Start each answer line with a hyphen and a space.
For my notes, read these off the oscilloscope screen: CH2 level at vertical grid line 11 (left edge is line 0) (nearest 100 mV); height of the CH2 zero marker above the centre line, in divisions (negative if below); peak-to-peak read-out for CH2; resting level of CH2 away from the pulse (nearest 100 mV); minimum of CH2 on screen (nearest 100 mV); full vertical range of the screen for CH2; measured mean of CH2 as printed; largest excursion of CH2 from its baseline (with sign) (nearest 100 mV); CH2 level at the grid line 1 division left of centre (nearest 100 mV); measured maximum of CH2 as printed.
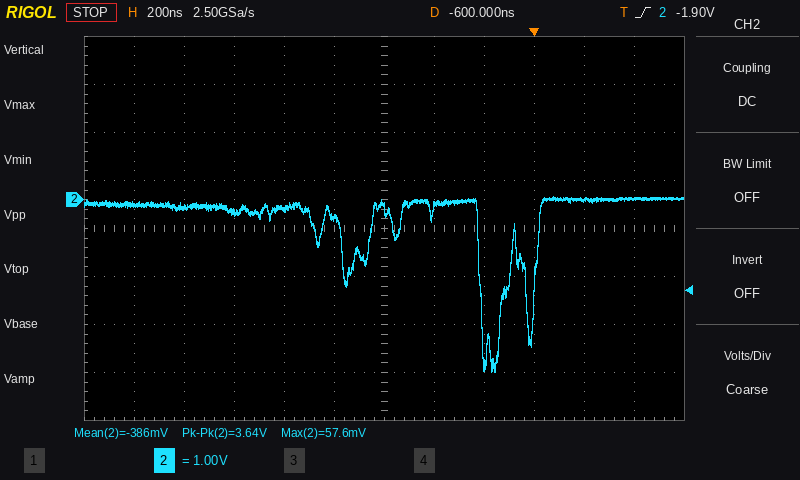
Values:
- 0.0 V
- +0.6 div
- 3.64 V
- -100 mV
- -3.6 V
- 8 V
- -386 mV
- -3.5 V
- -400 mV
- 57.6 mV
